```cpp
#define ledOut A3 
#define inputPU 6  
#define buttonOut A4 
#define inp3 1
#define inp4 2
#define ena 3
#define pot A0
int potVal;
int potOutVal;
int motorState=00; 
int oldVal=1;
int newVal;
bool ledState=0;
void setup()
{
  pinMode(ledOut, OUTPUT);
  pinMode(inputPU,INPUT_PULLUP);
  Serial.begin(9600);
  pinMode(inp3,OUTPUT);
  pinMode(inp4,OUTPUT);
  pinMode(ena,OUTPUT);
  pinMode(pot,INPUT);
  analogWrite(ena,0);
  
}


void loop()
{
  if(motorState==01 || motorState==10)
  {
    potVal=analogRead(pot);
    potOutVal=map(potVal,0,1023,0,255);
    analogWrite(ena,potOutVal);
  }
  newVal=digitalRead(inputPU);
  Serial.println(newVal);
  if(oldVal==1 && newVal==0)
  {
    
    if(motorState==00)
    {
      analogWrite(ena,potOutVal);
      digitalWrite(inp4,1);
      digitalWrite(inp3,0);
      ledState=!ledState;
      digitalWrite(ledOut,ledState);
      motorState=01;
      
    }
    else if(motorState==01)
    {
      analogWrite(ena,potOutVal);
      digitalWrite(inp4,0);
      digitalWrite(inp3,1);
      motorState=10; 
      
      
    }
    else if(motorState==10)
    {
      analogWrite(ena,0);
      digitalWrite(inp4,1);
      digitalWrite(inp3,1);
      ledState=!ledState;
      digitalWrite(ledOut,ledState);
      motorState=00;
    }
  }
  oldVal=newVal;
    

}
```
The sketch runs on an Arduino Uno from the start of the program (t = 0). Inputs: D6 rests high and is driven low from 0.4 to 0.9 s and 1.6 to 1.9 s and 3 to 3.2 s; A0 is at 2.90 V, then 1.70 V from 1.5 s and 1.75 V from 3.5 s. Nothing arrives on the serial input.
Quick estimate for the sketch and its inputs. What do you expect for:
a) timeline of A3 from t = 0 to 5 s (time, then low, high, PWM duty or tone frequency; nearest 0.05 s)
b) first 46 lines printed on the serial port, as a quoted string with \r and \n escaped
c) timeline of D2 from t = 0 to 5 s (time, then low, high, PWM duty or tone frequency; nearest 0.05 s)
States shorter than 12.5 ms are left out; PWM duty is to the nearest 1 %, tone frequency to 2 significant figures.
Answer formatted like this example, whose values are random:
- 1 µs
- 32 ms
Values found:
- 0 s low; 0.4 s high; 3 s low
- "1\r\n1\r\n1\r\n1\r\n1\r\n1\r\n1\r\n1\r\n1\r\n1\r\n1\r\n1\r\n1\r\n1\r\n1\r\n1\r\n1\r\n1\r\n1\r\n1\r\n1\r\n1\r\n1\r\n1\r\n1\r\n1\r\n1\r\n1\r\n1\r\n1\r\n1\r\n1\r\n1\r\n1\r\n1\r\n1\r\n1\r\n1\r\n1\r\n1\r\n1\r\n1\r\n1\r\n1\r\n1\r\n1\r\n"
- 0 s low; 0.4 s high; 1.6 s low; 3 s high
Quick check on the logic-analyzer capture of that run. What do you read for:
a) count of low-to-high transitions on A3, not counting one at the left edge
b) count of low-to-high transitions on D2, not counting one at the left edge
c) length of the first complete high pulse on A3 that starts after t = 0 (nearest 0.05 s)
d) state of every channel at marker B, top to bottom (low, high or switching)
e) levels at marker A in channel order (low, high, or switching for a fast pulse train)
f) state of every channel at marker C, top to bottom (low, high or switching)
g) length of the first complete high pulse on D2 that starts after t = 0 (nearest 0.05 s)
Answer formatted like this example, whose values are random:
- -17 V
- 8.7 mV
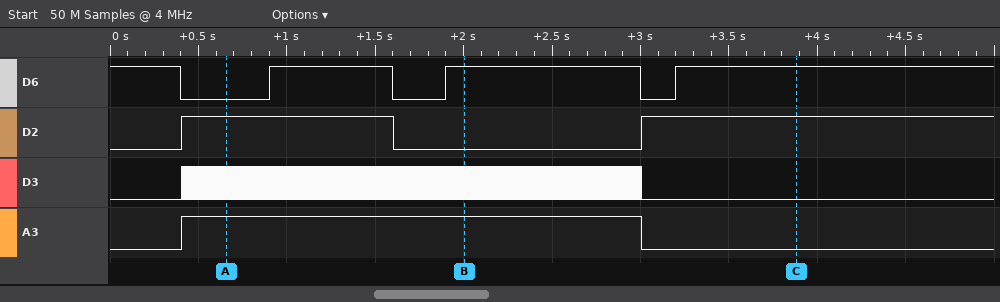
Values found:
- 1
- 2
- 2.60 s
- D6 high, D2 low, D3 switching, A3 high
- D6 low, D2 high, D3 switching, A3 high
- D6 high, D2 high, D3 low, A3 low
- 1.20 s
